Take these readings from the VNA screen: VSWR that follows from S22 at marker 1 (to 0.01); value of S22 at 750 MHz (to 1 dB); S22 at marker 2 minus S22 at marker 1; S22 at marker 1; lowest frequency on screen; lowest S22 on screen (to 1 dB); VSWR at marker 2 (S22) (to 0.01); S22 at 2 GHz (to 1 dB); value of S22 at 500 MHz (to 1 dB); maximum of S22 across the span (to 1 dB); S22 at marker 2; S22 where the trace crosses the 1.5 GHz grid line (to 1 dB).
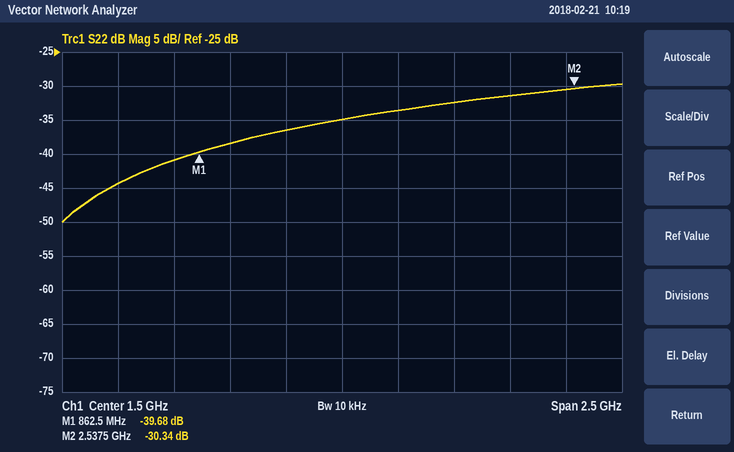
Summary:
1.02
-41 dB
9.34 dB
-39.68 dB
250 MHz
-50 dB
1.06
-32 dB
-44 dB
-30 dB
-30.34 dB
-35 dB
